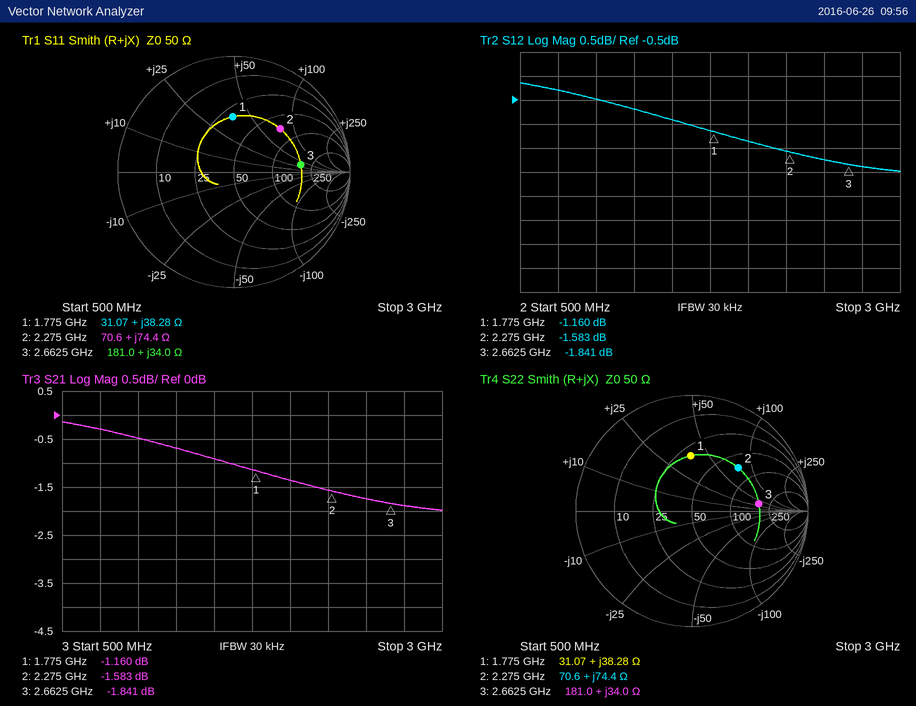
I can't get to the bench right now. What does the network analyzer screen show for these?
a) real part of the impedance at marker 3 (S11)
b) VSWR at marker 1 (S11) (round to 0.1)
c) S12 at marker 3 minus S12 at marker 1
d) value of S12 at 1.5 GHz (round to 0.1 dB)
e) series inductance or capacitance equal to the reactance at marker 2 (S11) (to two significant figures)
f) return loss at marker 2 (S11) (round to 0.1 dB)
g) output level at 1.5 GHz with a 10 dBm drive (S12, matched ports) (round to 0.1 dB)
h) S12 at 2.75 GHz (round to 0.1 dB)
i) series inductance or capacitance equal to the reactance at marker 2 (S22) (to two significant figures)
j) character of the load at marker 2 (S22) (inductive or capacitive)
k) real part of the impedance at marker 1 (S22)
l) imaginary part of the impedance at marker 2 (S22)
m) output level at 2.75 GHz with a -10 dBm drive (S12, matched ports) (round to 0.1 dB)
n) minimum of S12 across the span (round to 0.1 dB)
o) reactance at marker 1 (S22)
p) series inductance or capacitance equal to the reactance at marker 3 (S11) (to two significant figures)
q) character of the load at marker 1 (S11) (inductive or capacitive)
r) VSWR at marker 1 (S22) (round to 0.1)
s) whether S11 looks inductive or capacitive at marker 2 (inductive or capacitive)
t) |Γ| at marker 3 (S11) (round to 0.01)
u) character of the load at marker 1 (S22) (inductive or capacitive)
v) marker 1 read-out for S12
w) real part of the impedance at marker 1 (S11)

181.0 Ω
2.8
-0.681 dB
-0.9 dB
5.2 nH
5.3 dB
9.1 dBm
-1.9 dB
5.2 nH
inductive
31.07 Ω
+74.4 Ω
-11.9 dBm
-2.0 dB
+38.28 Ω
2.0 nH
inductive
2.8
inductive
0.58
inductive
-1.160 dB
31.07 Ω
